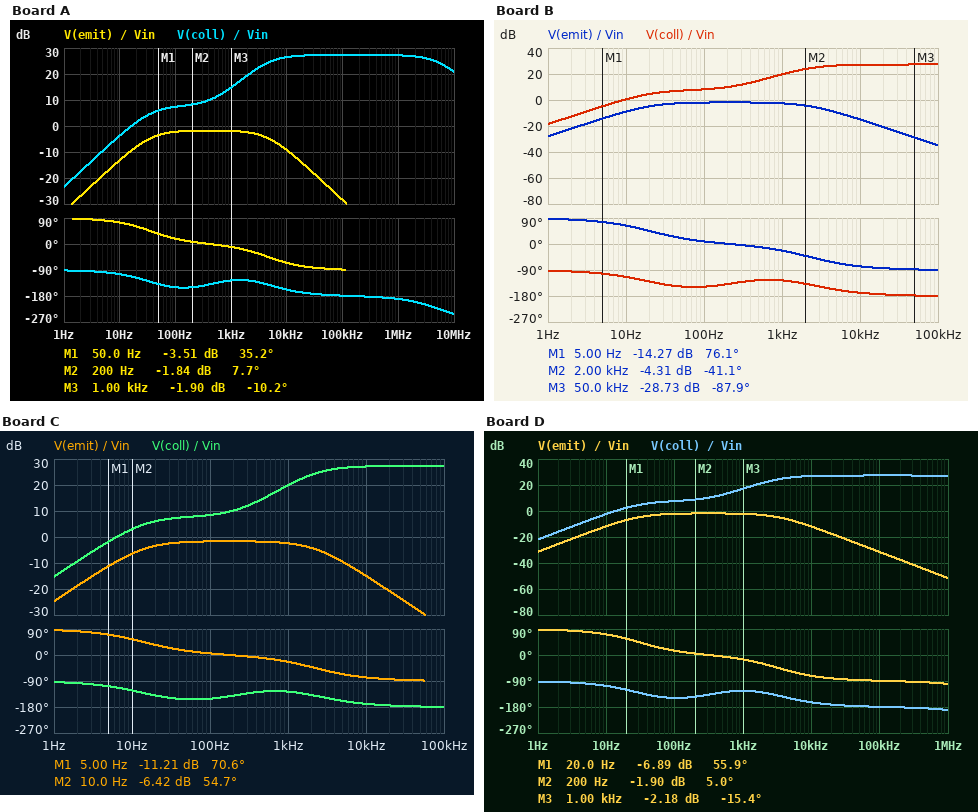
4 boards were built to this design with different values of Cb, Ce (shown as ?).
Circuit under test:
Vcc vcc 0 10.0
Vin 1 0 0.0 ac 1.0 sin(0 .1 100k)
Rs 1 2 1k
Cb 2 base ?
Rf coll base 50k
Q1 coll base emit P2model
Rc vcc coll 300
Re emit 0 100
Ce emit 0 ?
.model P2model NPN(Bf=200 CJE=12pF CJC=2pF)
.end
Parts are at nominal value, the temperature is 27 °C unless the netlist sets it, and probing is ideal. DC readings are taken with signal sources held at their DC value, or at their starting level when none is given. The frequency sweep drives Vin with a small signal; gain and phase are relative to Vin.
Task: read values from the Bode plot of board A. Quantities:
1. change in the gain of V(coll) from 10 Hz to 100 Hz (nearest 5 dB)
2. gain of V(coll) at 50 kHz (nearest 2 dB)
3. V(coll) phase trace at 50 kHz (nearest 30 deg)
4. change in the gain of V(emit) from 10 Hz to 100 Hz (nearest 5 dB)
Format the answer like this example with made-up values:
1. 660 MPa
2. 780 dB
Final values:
1. 10 dB
2. 28 dB
3. -180 deg
4. 10 dB
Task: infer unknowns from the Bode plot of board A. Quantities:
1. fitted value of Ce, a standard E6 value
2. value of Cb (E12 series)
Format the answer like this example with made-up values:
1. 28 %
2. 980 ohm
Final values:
1. 3.3 µF
2. 470 nF
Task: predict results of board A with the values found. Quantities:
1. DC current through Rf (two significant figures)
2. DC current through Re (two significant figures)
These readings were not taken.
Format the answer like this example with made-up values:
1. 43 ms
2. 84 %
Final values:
1. 70 µA
2. 14 mA
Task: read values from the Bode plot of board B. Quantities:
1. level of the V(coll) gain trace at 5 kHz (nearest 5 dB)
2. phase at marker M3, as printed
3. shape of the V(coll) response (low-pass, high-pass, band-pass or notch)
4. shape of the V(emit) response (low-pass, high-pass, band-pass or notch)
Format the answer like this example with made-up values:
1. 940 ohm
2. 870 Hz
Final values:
1. 25 dB
2. -87.9 deg
3. high-pass
4. band-pass
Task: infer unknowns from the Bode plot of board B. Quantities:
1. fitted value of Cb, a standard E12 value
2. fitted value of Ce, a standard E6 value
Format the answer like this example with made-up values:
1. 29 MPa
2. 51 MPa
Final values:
1. 820 nF
2. 6.8 µF
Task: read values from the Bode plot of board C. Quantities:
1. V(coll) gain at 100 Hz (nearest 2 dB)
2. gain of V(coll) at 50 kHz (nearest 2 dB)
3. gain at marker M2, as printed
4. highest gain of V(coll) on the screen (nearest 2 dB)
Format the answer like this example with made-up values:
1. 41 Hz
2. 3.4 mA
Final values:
1. 8 dB
2. 28 dB
3. -6.42 dB
4. 28 dB
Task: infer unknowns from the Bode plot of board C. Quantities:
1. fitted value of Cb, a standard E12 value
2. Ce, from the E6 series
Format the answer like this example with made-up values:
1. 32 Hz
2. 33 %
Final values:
1. 1.2 µF
2. 6.8 µF
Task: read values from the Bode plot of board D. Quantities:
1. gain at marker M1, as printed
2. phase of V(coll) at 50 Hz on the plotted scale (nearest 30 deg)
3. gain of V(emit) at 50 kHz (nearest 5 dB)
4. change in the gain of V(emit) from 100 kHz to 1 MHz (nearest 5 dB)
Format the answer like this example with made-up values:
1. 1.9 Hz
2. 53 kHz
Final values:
1. -6.89 dB
2. -150 deg
3. -25 dB
4. -20 dB
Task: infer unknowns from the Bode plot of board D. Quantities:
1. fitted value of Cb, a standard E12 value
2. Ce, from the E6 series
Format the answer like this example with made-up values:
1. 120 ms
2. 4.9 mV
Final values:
1. 560 nF
2. 4.7 µF
